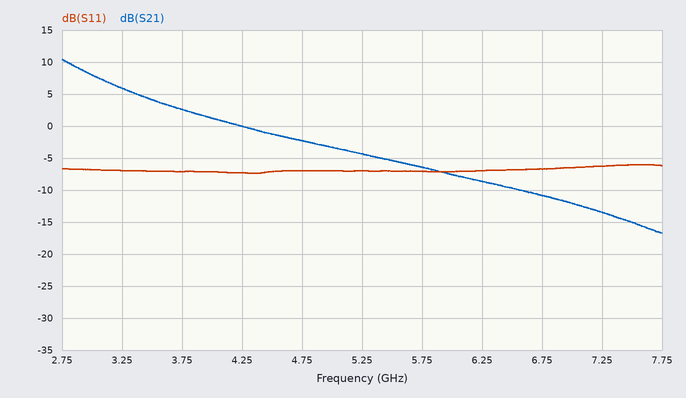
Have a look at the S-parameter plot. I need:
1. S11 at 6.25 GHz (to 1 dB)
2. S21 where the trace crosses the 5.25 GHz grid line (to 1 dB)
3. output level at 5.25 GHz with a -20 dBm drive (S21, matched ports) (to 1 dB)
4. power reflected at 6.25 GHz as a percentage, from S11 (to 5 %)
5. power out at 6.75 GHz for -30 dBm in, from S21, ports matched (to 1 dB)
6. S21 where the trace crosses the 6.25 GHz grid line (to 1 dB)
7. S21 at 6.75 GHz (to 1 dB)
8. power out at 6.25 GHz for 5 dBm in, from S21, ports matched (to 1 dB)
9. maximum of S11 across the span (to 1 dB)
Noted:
-7 dB
-4 dB
-24 dBm
20 %
-41 dBm
-9 dB
-11 dB
-4 dBm
-6 dB
